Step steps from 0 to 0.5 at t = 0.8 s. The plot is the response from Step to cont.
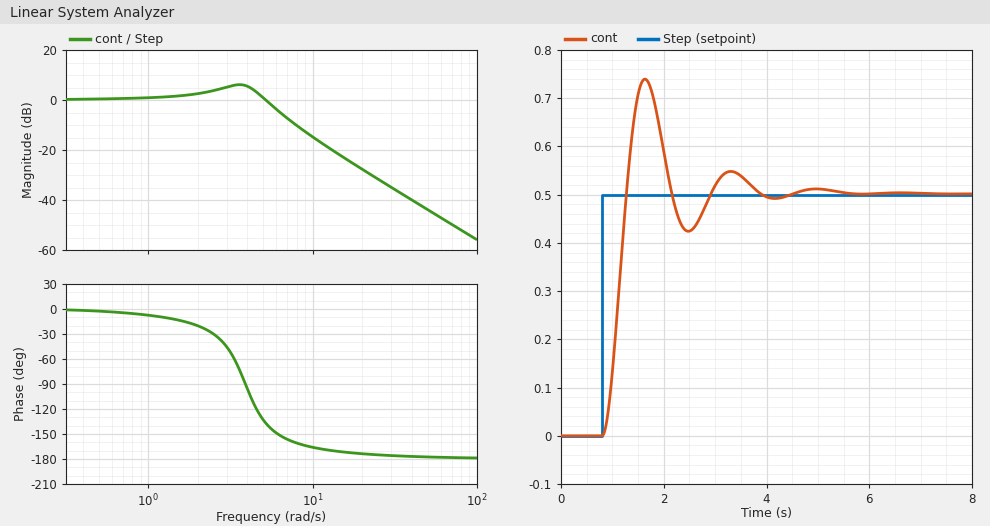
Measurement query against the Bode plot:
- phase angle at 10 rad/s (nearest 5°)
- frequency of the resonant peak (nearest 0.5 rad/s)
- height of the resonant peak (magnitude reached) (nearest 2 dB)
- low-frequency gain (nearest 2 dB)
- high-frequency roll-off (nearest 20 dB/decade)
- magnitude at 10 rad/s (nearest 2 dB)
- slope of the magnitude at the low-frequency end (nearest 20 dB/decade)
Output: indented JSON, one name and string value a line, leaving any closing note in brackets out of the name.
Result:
{
  "phase angle at 10 rad/s": "-165°",
  "frequency of the resonant peak": "3.5 rad/s",
  "height of the resonant peak (magnitude reached)": "6 dB",
  "low-frequency gain": "0 dB",
  "high-frequency roll-off": "-40 dB/decade",
  "magnitude at 10 rad/s": "-14 dB",
  "slope of the magnitude at the low-frequency end": "0 dB/decade"
}
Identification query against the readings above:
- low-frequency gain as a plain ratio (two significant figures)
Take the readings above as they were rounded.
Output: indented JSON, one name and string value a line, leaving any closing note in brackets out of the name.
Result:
{
  "low-frequency gain as a plain ratio": "1.0"
}
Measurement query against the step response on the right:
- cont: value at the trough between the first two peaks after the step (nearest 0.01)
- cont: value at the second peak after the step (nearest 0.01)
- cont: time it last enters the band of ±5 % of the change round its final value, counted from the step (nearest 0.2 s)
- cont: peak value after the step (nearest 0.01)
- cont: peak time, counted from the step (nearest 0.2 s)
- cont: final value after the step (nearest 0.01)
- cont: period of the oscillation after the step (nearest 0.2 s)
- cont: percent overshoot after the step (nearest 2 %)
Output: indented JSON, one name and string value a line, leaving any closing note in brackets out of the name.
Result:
{
  "cont: value at the trough between the first two peaks after the step": "0.42",
  "cont: value at the second peak after the step": "0.55",
  "cont: time it last enters the band of ±5 % of the change round its final value, counted from the step": "2.8 s",
  "cont: peak value after the step": "0.74",
  "cont: peak time, counted from the step": "0.8 s",
  "cont: final value after the step": "0.50",
  "cont: period of the oscillation after the step": "1.6 s",
  "cont: percent overshoot after the step": "48 %"
}
